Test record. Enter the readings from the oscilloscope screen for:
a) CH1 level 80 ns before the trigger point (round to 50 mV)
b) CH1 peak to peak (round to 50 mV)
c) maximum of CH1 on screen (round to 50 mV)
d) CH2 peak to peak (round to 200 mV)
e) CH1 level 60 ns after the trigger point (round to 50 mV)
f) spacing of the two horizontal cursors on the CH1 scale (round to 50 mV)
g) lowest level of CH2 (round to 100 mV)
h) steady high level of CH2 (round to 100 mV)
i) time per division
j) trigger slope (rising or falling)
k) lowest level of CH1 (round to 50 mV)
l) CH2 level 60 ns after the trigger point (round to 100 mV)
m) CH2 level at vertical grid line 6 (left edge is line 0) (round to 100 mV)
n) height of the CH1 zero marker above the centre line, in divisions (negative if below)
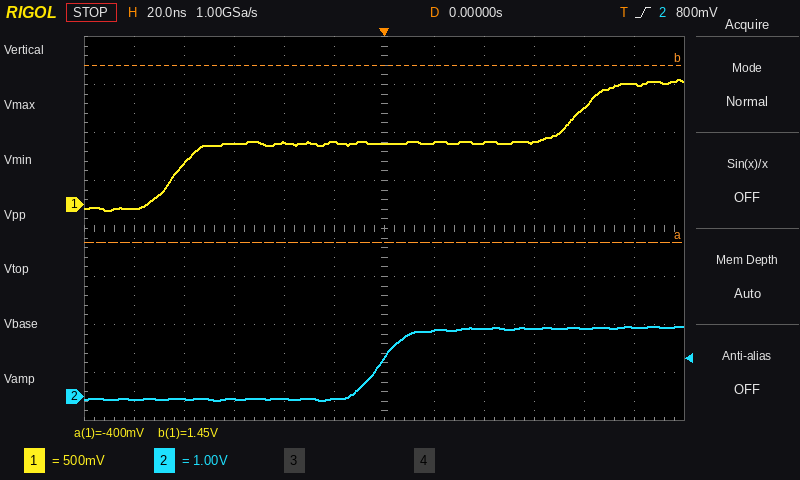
450 mV
1.35 V
1.30 V
1.6 V
650 mV
1.85 V
-100 mV
1.4 V
20 ns
rising
-50 mV
1.4 V
800 mV
+0.5 div
